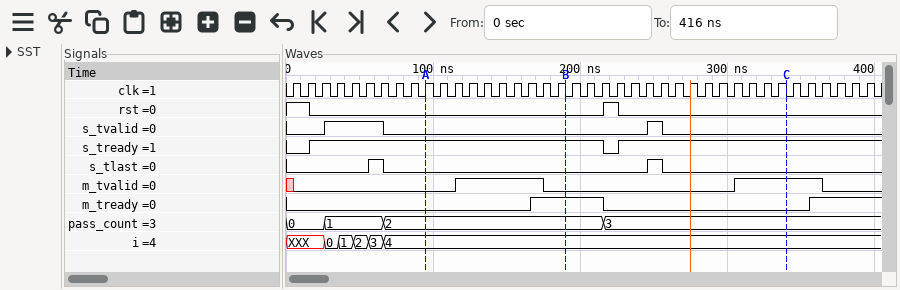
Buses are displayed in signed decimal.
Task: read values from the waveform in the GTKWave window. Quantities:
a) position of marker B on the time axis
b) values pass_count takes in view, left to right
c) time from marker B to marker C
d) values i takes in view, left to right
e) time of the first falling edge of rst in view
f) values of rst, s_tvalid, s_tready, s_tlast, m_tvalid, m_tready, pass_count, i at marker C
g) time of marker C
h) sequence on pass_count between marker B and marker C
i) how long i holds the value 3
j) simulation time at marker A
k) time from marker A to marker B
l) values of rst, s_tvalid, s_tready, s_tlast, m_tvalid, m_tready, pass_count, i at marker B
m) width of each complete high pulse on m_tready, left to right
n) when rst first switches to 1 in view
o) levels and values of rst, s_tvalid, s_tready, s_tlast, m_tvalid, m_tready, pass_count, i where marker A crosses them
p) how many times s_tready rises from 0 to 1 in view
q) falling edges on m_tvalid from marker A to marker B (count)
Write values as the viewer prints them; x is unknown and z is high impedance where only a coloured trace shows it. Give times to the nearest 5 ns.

190 ns
0, 1, 2, 3
150 ns
XXX, 0, 1, 2, 3, 4
15 ns
rst=0, s_tvalid=0, s_tready=1, s_tlast=0, m_tvalid=1, m_tready=0, pass_count=3, i=4
340 ns
2, 3
10 ns
95 ns
95 ns
rst=0, s_tvalid=0, s_tready=1, s_tlast=0, m_tvalid=0, m_tready=1, pass_count=2, i=4
50 ns
215 ns
rst=0, s_tvalid=0, s_tready=1, s_tlast=0, m_tvalid=0, m_tready=0, pass_count=2, i=4
2
1
